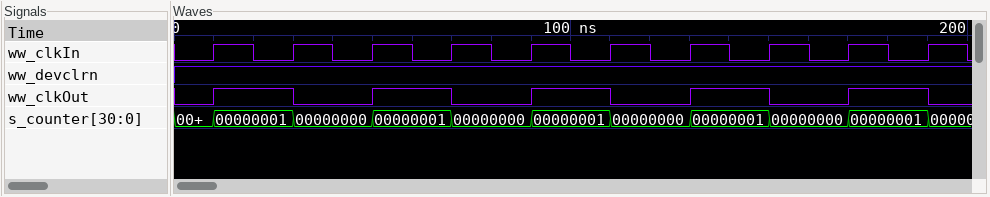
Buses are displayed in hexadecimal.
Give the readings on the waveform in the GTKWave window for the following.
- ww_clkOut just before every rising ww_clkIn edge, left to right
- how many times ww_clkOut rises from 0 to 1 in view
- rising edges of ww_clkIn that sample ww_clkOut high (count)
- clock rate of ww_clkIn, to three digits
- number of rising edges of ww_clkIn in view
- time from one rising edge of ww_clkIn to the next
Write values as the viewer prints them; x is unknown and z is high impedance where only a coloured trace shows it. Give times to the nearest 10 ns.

0 1 0 1 0 1 0 1 0 1
5
5
50.0 MHz
10
20 ns
